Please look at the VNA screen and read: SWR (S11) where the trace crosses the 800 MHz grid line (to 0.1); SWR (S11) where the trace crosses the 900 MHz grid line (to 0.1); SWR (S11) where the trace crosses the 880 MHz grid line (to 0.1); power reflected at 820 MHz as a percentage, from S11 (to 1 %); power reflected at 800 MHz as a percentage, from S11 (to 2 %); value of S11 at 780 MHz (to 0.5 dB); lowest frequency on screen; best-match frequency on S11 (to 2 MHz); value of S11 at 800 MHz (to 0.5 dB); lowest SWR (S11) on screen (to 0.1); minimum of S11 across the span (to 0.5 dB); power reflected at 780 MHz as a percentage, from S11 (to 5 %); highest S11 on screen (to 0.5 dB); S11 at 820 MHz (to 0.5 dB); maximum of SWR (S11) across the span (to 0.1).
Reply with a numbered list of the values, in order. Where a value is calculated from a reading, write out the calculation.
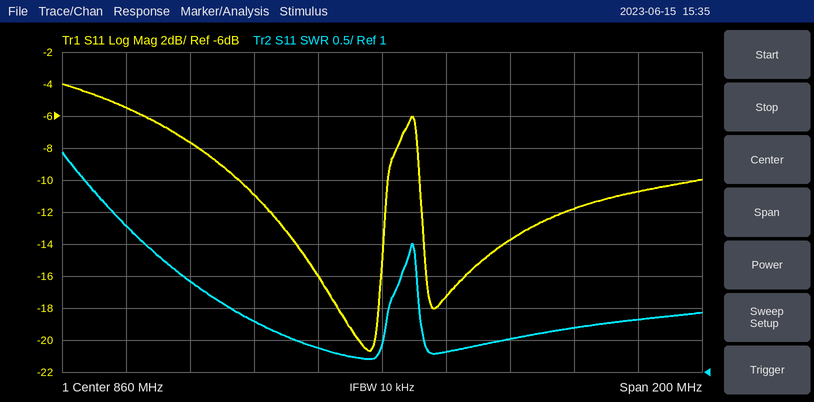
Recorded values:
1. 2.4
2. 1.5
3. 1.3
4. 10^(-11/10) ≈ 8 %
5. 10^(-7.5/10) ≈ 18 %
6. -5.5 dB
7. 760 MHz
8. 856 MHz
9. -7.5 dB
10. 1.2
11. -20.5 dB
12. 10^(-5.5/10) ≈ 28.2 %, so 30 % to the nearest 5 %
13. -4.0 dB
14. -11.0 dB
15. 4.4
